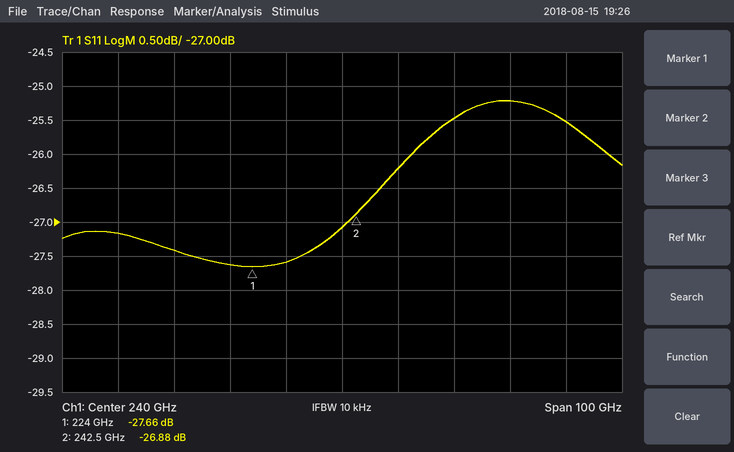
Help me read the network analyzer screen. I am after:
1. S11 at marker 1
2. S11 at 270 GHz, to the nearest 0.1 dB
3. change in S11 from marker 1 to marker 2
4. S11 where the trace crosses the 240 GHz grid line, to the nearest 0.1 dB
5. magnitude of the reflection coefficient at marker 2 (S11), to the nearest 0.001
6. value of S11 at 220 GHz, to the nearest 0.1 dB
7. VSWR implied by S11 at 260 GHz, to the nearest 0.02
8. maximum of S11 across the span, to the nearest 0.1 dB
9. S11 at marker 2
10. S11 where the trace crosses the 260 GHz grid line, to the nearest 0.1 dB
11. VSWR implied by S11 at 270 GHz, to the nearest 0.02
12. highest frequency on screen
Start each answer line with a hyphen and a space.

- -27.66 dB
- -25.2 dB
- 0.78 dB
- -27.1 dB
- 0.045
- -27.6 dB
- 1.12
- -25.2 dB
- -26.88 dB
- -25.5 dB
- 1.12
- 290 GHz
